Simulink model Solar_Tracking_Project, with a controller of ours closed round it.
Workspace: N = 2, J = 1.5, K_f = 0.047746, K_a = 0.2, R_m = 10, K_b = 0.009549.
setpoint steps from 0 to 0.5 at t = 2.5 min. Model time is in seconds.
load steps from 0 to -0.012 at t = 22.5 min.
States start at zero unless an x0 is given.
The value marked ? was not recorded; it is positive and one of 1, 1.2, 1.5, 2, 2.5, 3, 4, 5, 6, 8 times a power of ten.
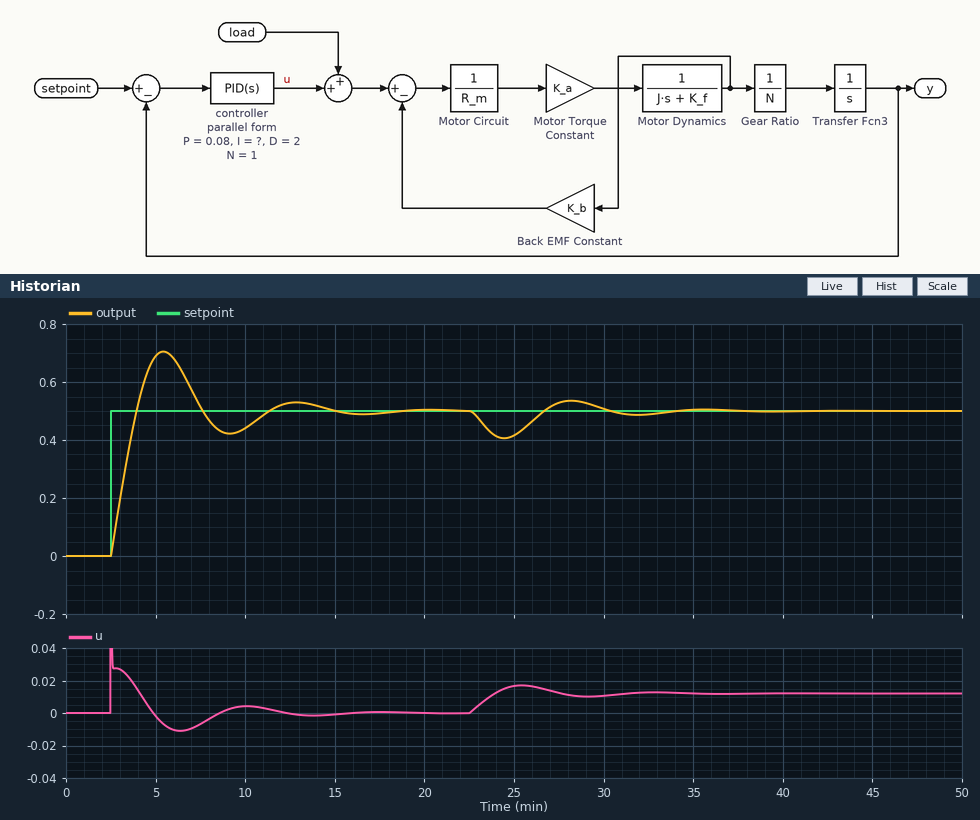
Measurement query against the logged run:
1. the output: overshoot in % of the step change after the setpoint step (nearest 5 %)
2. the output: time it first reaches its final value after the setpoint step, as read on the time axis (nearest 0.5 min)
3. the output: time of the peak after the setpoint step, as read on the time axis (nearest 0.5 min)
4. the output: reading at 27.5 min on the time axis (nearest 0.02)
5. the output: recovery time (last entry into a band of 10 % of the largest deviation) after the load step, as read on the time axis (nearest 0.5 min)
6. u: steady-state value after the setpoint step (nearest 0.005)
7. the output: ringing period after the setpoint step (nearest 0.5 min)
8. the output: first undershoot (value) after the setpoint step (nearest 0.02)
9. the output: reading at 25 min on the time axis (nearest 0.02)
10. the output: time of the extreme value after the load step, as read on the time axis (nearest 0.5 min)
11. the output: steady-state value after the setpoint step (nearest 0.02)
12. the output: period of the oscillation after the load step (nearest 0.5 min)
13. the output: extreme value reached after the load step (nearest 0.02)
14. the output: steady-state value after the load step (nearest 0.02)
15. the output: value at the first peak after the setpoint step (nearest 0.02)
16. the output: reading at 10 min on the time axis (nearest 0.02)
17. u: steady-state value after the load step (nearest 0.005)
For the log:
40 %
4.0 min
5.5 min
0.52
33.0 min
0.000
7.5 min
0.42
0.42
24.5 min
0.50
7.5 min
0.40
0.50
0.70
0.44
0.010
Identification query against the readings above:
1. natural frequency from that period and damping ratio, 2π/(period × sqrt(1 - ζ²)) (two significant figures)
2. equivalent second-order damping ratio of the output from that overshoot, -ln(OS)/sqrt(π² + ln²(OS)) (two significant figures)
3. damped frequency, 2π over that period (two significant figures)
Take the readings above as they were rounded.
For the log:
0.87 rad/min
0.28
0.84 rad/min
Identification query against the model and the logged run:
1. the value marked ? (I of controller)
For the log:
0.0012
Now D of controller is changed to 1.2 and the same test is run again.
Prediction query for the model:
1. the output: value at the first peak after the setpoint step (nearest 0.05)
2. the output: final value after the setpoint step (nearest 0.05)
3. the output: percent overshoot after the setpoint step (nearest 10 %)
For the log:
0.75
0.50
50 %
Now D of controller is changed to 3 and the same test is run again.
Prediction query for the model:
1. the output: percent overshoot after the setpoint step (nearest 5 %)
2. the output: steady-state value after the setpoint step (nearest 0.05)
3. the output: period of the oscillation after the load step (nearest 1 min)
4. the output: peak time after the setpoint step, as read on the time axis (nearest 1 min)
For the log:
35 %
0.50
8 min
6 min
